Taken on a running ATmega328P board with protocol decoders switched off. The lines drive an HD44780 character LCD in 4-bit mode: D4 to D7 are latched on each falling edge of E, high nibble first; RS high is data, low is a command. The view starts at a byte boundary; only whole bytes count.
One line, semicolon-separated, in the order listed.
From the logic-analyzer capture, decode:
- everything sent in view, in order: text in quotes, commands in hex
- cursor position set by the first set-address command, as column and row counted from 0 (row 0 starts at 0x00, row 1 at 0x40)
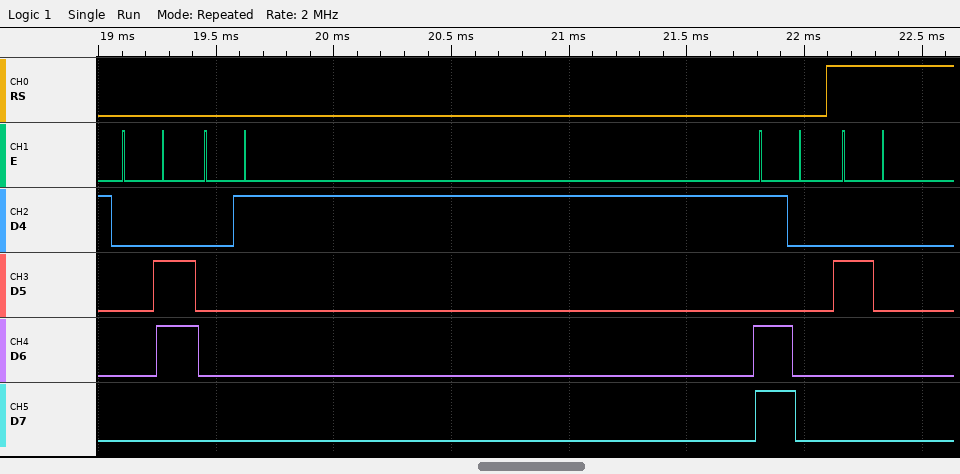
0x06 0x01 0xD0 " "; column 16, row 1
